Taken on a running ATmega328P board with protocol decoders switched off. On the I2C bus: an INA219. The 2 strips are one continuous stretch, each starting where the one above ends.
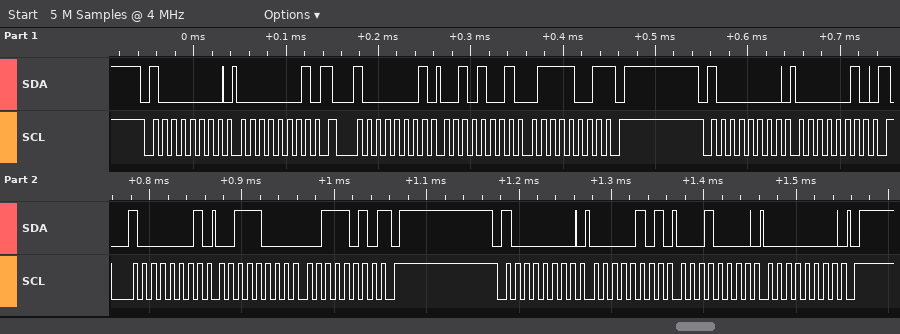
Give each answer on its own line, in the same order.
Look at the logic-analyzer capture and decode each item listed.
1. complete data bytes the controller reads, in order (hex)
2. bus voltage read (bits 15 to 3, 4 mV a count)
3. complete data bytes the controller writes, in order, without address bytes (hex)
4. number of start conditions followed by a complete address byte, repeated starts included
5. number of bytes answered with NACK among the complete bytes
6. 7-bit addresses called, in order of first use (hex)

29 79 38 3A
7.196 V
01 02 05 10 00
5
2
0x40
